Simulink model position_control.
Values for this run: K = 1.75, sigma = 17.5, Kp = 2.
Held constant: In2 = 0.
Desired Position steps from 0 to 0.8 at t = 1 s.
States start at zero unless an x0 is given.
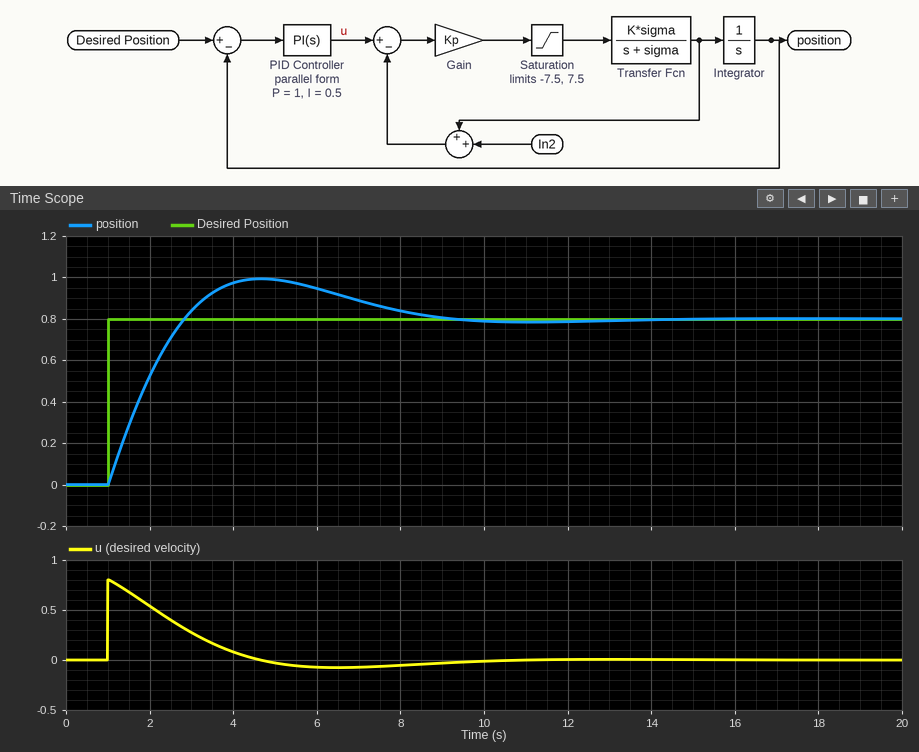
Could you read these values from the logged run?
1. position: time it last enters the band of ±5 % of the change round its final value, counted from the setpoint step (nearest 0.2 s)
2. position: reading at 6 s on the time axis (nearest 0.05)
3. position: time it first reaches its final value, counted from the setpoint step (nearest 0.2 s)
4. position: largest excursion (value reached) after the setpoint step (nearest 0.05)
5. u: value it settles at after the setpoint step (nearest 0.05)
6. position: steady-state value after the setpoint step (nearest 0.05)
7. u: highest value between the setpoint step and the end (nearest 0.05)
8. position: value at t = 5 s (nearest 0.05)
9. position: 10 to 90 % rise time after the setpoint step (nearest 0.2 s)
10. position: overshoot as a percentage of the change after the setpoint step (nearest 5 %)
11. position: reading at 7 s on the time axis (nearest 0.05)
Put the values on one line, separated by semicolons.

7.0 s; 0.95; 1.8 s; 1.00; 0.00; 0.80; 0.80; 1.00; 1.4 s; 25 %; 0.90
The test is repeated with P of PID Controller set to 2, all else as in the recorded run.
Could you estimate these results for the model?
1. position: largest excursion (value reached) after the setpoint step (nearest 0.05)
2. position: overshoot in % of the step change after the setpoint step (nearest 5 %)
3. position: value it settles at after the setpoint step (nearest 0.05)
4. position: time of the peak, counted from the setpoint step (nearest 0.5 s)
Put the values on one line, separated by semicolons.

0.90; 10 %; 0.80; 3.0 s
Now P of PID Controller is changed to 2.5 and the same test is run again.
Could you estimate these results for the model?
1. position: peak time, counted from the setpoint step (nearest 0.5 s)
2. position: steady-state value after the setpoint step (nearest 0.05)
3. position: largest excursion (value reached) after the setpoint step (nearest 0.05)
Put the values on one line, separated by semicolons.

2.5 s; 0.80; 0.85
